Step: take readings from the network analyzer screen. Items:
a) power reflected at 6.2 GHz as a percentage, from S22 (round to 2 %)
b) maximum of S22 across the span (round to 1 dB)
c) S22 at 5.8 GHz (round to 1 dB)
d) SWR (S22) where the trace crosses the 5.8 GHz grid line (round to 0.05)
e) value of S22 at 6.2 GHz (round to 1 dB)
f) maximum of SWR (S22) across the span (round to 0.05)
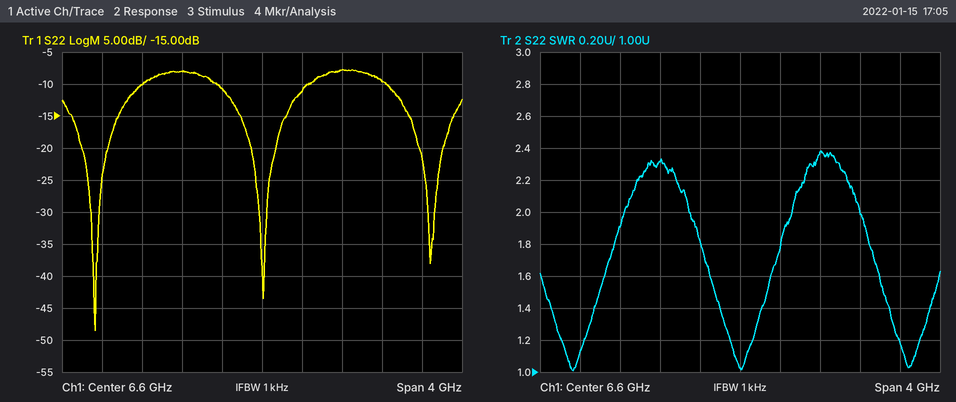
8 %
-8 dB
-8 dB
2.30
-11 dB
2.40
